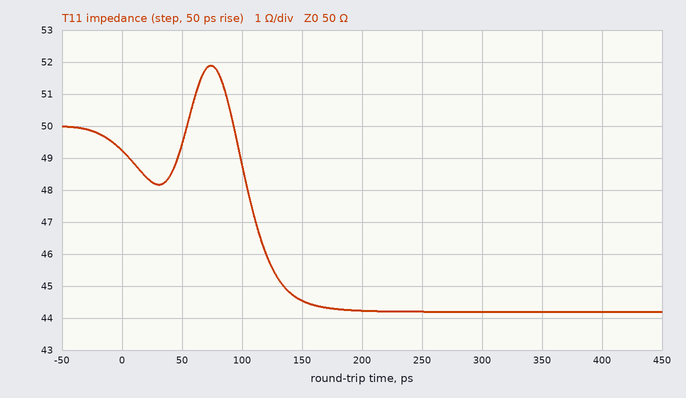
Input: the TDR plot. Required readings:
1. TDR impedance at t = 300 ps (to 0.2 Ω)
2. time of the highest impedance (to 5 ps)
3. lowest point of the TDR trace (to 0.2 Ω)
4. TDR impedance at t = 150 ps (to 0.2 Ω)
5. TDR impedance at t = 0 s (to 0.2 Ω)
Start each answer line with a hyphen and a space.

- 44.2 Ω
- 75 ps
- 44.2 Ω
- 44.6 Ω
- 49.2 Ω
